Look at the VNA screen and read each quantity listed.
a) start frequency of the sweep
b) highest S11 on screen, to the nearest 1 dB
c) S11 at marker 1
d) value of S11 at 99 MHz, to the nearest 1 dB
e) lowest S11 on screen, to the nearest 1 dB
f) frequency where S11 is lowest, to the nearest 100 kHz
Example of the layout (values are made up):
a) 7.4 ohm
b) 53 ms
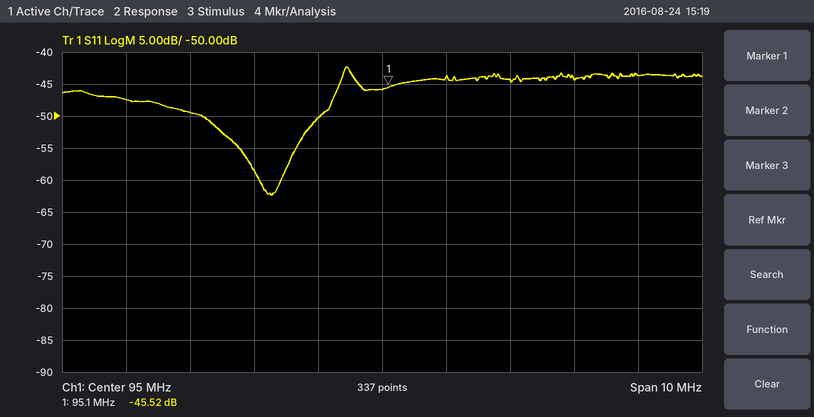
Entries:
a) 90 MHz
b) -42 dB
c) -45.52 dB
d) -44 dB
e) -62 dB
f) 93.3 MHz
